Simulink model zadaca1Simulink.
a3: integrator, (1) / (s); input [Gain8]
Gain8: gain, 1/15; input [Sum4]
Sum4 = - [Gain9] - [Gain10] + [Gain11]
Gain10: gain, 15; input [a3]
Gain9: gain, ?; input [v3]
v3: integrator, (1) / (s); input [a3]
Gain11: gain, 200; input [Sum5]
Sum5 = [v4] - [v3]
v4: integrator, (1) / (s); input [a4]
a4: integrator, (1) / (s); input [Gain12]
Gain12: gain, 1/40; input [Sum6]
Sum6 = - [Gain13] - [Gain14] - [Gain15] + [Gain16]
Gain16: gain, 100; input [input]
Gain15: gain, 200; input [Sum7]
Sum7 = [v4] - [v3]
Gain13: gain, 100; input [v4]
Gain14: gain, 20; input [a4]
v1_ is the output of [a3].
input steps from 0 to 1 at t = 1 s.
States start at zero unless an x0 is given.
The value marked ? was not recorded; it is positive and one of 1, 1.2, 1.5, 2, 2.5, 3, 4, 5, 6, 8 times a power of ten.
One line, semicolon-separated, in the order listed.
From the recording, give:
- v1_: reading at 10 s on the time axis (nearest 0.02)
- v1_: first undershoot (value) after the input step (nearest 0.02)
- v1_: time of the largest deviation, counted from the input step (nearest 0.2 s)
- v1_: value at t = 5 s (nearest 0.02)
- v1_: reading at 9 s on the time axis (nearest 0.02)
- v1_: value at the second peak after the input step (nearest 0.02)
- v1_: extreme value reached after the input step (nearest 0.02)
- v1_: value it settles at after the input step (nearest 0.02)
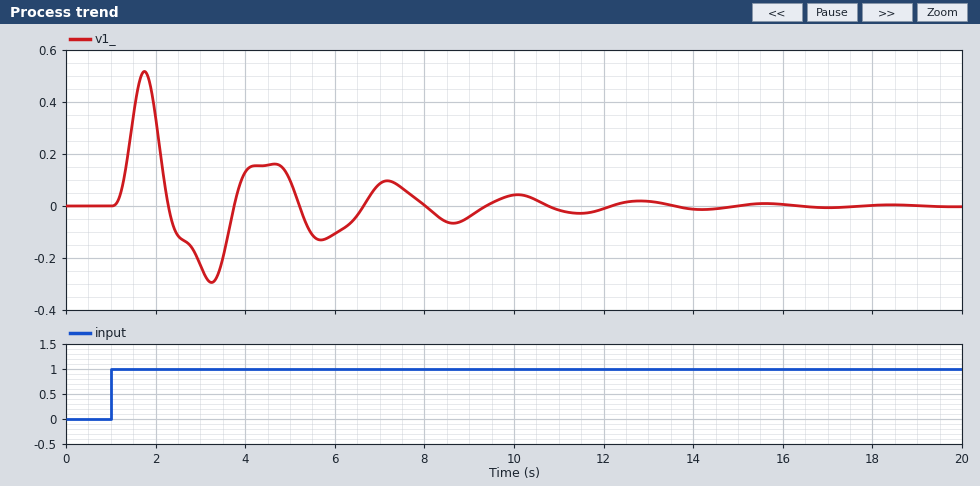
0.04; -0.30; 0.8 s; 0.10; -0.04; 0.16; 0.52; 0.00
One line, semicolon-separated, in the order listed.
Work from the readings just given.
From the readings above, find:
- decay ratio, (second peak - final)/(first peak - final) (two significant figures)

0.31
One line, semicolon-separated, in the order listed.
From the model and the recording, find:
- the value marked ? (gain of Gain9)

300
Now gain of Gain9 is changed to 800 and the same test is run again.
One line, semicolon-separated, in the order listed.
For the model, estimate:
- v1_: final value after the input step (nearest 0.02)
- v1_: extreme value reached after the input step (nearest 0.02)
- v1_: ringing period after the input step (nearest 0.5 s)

0.00; 0.24; 2.5 s
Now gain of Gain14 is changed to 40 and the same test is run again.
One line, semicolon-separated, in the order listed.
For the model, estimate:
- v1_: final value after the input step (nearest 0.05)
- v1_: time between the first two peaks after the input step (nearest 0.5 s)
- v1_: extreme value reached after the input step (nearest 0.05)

0.00; 3.0 s; 0.45
